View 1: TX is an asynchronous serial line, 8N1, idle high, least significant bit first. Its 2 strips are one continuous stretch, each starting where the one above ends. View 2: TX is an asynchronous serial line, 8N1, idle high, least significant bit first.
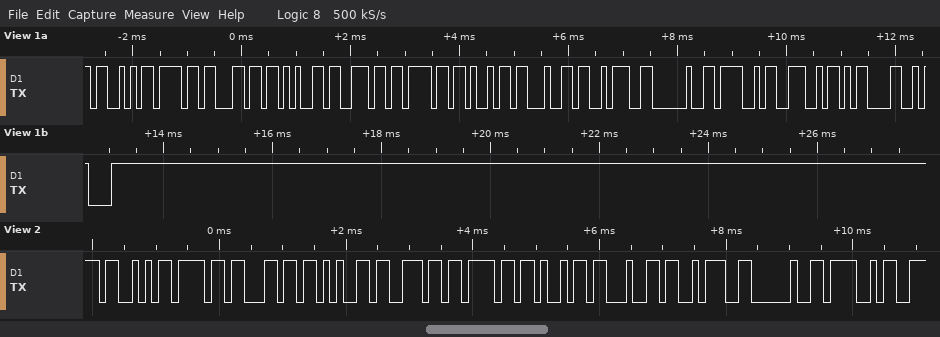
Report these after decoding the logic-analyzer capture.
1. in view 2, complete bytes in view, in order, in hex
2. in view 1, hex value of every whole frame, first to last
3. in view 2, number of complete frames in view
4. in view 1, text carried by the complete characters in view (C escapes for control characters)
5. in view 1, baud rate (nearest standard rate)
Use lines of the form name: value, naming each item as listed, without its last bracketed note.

in view 2, complete bytes in view, in order, in hex: 53 6F 6C 65 6E 6F 69 64 3A 20 4F
in view 1, hex value of every whole frame, first to last: 53 6F 6C 65 6E 6F 69 64 3A 20 4F 4E 0D 0A
in view 2, number of complete frames in view: 11
in view 1, text carried by the complete characters in view: "Solenoid: ON\r\n"
in view 1, baud rate: 9600 baud
